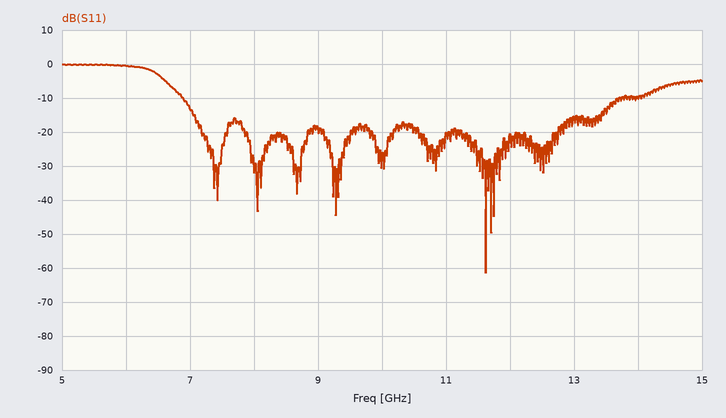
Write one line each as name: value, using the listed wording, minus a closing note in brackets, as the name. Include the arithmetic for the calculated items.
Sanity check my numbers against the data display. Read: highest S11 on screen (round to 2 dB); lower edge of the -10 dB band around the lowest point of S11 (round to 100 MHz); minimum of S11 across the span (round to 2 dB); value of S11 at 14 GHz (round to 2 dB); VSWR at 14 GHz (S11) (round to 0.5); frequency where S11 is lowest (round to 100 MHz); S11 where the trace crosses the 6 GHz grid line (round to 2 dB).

highest S11 on screen: 0 dB
lower edge of the -10 dB band around the lowest point of S11: 6.9 GHz
minimum of S11 across the span: -62 dB
value of S11 at 14 GHz: -10 dB
VSWR at 14 GHz (S11): |Γ| = 10^(-10/20) = 0.3162; VSWR = (1 + 0.3162)/(1 − 0.3162) ≈ 1.92, so 2.0 to the nearest 0.5
frequency where S11 is lowest: 11.6 GHz
S11 where the trace crosses the 6 GHz grid line: 0 dB
